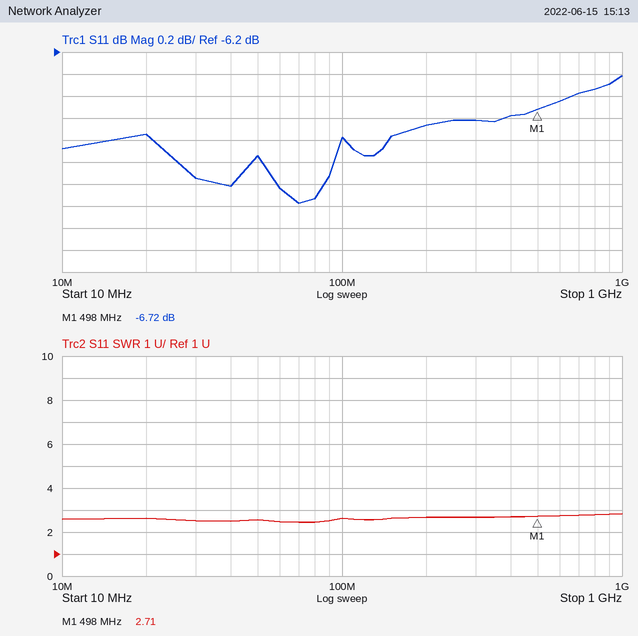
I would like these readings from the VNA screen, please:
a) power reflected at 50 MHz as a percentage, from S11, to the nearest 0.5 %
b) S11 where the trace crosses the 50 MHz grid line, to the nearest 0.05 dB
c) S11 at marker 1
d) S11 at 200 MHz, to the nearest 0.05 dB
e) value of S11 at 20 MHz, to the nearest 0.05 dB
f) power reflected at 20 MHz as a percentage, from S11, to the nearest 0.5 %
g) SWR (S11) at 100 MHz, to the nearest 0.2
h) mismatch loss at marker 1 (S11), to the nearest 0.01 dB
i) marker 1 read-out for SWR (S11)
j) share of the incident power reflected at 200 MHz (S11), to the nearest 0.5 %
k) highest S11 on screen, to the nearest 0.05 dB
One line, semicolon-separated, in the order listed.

19.5 %; -7.15 dB; -6.72 dB; -6.85 dB; -6.95 dB; 20.0 %; 2.6; 1.04 dB; 2.71; 20.5 %; -6.40 dB
